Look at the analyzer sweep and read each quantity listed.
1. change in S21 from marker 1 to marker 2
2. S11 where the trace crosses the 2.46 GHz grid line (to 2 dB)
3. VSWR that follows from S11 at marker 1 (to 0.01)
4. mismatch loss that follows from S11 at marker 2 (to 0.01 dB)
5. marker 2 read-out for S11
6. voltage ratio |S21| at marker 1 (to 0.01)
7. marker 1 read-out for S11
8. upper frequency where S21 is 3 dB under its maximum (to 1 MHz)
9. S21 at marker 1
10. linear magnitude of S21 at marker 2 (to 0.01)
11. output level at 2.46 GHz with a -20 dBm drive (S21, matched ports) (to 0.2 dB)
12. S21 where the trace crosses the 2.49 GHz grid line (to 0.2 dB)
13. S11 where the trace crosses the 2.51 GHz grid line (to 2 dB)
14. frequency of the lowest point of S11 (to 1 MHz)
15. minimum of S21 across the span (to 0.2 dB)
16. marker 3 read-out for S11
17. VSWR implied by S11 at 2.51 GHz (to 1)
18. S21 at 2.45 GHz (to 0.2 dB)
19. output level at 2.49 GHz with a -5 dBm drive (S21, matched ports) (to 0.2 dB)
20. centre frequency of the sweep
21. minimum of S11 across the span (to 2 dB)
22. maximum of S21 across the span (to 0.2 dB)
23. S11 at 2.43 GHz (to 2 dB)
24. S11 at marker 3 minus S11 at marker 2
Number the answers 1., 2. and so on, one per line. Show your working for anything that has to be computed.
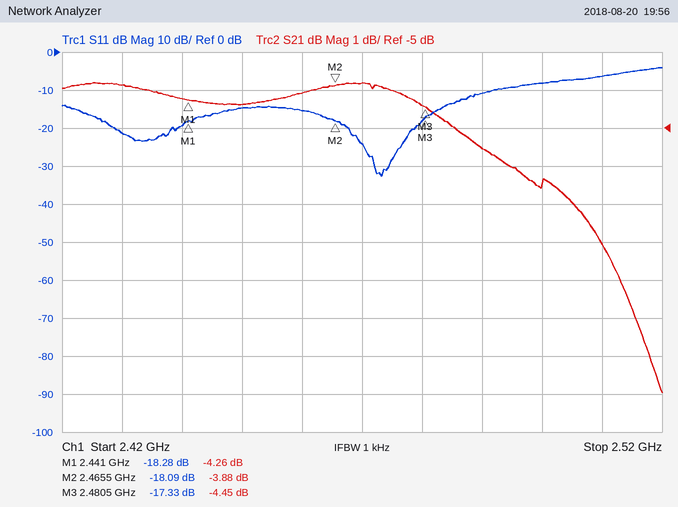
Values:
1. -3.88 − (-4.26) = 0.38 dB
2. -16 dB
3. (1 + 0.1219)/(1 − 0.1219) ≈ 1.28
4. −10 log10(1 − 10^(-18.09/10)) ≈ 0.07 dB
5. -18.09 dB
6. 10^(-4.26/20) ≈ 0.61
7. -18.28 dB
8. 2.504 GHz
9. -4.26 dB
10. 10^(-3.88/20) ≈ 0.64
11. -20 dBm + (-4.0 dB) = -24.0 dBm
12. -5.6 dB
13. -6 dB
14. 2.473 GHz
15. -12.0 dB
16. -17.33 dB
17. |Γ| = 10^(-6/20) = 0.5012; VSWR = (1 + 0.5012)/(1 − 0.5012) ≈ 3
18. -4.4 dB
19. -5 dBm + (-5.6 dB) = -10.6 dBm
20. 2.47 GHz
21. -32 dB
22. -3.8 dB
23. -22 dB
24. -17.33 − (-18.09) = 0.76 dB
